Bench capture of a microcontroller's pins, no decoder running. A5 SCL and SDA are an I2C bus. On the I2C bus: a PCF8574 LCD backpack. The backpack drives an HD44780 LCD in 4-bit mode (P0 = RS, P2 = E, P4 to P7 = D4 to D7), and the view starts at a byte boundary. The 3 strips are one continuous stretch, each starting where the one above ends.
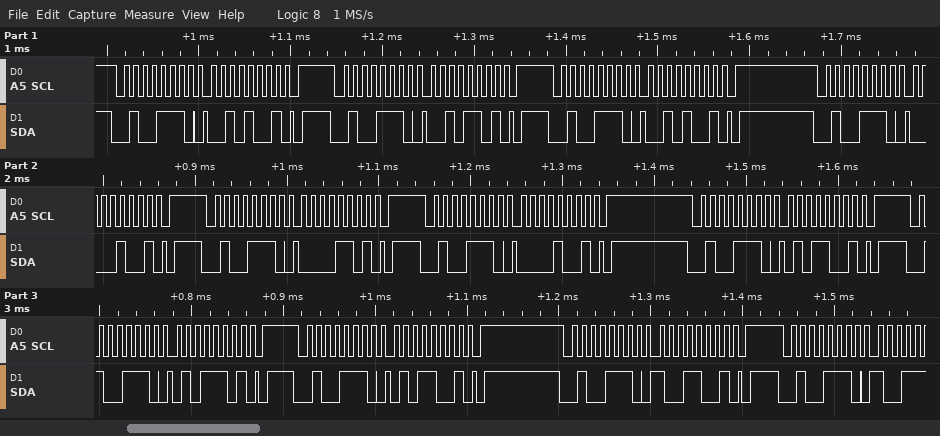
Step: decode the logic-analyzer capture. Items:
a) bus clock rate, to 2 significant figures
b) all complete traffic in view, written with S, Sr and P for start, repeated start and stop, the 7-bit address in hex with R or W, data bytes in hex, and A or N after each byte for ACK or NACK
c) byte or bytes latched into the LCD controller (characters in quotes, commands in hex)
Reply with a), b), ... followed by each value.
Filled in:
a) 100 kHz
b) S 27W A 29 A P S 27W A 2D A P S 27W A 29 A P S 27W A 09 A P S 27W A 0D A P S 27W A 09 A P S 27W A 59 A P S 27W A 5D A P S 27W A 59 A P S 27W A 99 A P S 27W A
c) ' '
